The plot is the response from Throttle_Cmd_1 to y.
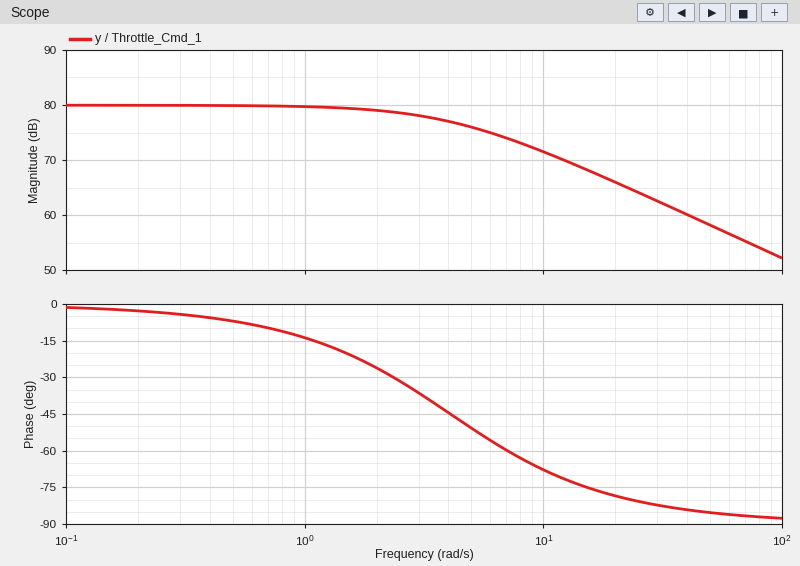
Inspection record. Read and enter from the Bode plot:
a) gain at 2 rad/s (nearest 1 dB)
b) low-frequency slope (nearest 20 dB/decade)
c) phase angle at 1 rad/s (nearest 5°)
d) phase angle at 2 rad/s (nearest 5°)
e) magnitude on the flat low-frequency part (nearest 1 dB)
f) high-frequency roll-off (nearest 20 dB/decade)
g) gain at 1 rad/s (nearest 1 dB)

79 dB
0 dB/decade
-15°
-25°
80 dB
-20 dB/decade
80 dB
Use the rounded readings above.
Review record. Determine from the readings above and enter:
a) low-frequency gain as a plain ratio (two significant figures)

10000
